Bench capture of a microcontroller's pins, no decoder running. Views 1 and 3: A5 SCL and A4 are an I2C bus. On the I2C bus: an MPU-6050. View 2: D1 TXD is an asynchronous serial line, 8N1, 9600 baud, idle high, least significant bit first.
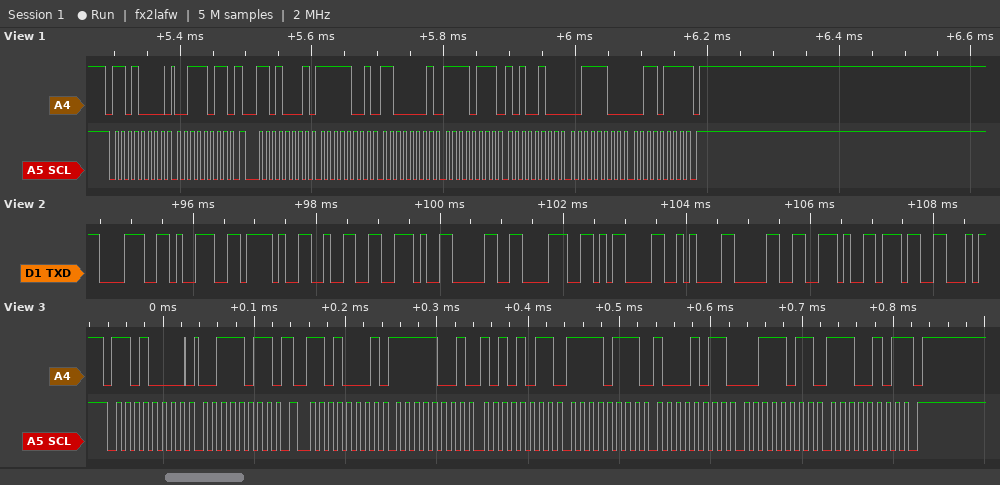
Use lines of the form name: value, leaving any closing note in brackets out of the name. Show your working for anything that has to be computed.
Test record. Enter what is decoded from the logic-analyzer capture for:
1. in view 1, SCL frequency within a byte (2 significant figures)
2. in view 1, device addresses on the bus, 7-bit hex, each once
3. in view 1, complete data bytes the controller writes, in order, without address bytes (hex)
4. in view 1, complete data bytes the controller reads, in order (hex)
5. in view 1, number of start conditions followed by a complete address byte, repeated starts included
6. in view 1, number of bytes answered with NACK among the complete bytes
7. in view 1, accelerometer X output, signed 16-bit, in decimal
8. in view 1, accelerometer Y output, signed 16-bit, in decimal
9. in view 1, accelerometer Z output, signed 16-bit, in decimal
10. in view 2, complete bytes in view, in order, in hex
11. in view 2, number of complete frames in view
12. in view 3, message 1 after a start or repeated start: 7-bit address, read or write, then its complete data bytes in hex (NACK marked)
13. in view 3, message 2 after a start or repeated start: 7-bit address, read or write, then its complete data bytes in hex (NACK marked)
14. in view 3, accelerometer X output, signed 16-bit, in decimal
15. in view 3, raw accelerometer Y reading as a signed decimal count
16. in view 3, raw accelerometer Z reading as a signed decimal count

in view 1, SCL frequency within a byte: 100 kHz
in view 1, device addresses on the bus, 7-bit hex, each once: 0x68
in view 1, complete data bytes the controller writes, in order, without address bytes: 3B
in view 1, complete data bytes the controller reads, in order: F9 C1 F7 A4 3C 37
in view 1, number of start conditions followed by a complete address byte, repeated starts included: 2
in view 1, number of bytes answered with NACK among the complete bytes: 1
in view 1, accelerometer X output, signed 16-bit, in decimal: 0xF9C1 = -1599
in view 1, accelerometer Y output, signed 16-bit, in decimal: 0xF7A4 = -2140
in view 1, accelerometer Z output, signed 16-bit, in decimal: 0x3C37 = 15415
in view 2, complete bytes in view, in order, in hex: 38 39 2F 32 2E 30 38 0D 0A 30 2E 37
in view 2, number of complete frames in view: 12
in view 3, message 1 after a start or repeated start: 7-bit address, read or write, then its complete data bytes in hex: 0x68 write: 3B
in view 3, message 2 after a start or repeated start: 7-bit address, read or write, then its complete data bytes in hex: 0x68 read: F9 AB F7 8B 3B E5 NACK
in view 3, accelerometer X output, signed 16-bit, in decimal: 0xF9AB = -1621
in view 3, raw accelerometer Y reading as a signed decimal count: 0xF78B = -2165
in view 3, raw accelerometer Z reading as a signed decimal count: 0x3BE5 = 15333
